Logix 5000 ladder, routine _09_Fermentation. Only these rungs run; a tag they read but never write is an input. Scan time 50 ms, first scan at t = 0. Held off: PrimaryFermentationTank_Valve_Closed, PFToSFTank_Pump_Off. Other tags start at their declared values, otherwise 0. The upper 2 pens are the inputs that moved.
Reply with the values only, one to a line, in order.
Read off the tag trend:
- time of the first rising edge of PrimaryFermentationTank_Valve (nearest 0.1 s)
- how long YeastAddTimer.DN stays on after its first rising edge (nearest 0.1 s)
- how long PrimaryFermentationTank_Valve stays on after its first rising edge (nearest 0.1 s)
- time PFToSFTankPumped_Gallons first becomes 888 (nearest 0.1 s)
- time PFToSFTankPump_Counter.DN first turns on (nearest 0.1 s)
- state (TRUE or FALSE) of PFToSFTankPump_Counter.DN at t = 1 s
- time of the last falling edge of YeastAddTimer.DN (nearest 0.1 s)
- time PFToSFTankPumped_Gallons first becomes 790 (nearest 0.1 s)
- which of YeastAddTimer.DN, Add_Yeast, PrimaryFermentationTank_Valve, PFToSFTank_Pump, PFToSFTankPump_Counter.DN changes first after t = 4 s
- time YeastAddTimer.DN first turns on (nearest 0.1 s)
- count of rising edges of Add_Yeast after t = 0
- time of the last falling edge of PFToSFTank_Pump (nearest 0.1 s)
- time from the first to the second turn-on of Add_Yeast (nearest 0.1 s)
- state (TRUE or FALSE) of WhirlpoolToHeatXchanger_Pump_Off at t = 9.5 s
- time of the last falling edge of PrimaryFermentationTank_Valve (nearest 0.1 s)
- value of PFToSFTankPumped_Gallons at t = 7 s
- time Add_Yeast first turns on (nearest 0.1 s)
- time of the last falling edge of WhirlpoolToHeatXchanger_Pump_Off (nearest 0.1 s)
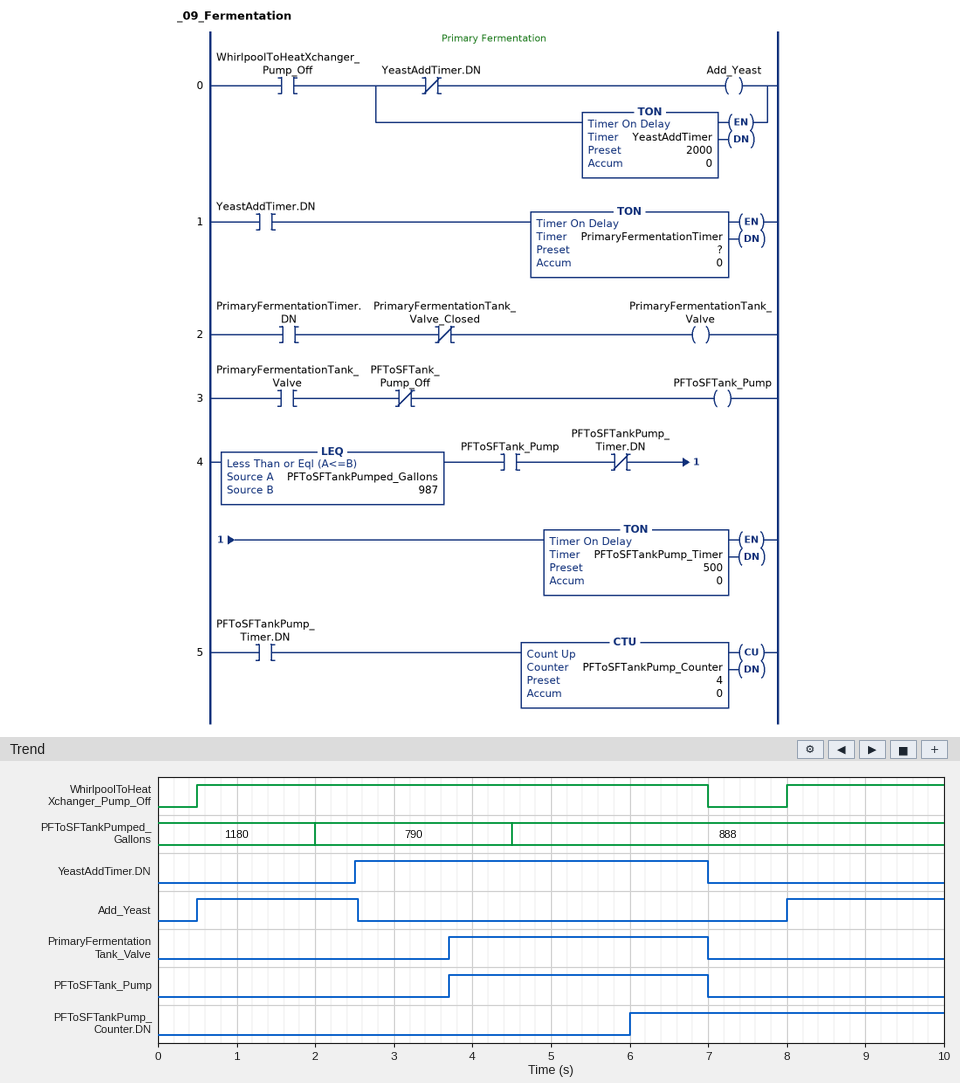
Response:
3.7 s
4.5 s
3.3 s
4.5 s
6.0 s
FALSE
7.0 s
2.0 s
PFToSFTankPump_Counter.DN
2.5 s
2
7.0 s
7.5 s
TRUE
7.0 s
888
0.5 s
7.0 s
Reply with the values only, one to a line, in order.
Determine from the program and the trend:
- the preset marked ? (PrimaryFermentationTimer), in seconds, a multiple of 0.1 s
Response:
1.2 s
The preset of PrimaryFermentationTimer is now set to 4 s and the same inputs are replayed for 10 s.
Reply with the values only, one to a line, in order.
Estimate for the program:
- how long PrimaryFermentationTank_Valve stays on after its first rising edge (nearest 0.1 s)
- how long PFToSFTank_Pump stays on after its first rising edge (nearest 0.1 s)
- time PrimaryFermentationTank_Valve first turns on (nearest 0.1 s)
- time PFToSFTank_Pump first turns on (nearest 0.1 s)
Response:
0.5 s
0.5 s
6.5 s
6.5 s
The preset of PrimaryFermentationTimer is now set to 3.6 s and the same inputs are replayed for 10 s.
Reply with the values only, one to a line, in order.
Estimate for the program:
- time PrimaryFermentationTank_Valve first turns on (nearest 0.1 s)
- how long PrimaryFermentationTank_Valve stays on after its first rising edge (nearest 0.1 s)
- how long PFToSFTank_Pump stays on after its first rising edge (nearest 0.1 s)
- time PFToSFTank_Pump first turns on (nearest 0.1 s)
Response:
6.1 s
0.9 s
0.9 s
6.1 s
